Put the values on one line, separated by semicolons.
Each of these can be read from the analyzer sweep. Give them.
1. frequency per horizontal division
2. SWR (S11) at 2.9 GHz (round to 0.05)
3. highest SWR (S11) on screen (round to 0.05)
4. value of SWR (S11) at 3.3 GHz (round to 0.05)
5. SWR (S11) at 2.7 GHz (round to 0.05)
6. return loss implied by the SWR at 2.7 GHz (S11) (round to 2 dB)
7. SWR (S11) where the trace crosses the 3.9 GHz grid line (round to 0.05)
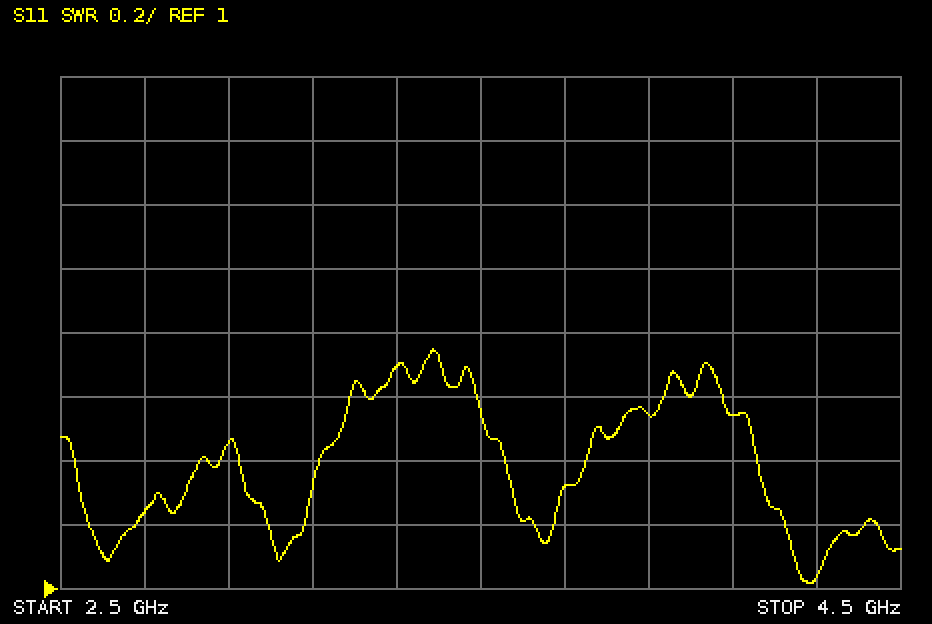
200 MHz; 1.45; 1.75; 1.70; 1.25; 20 dB; 1.55
